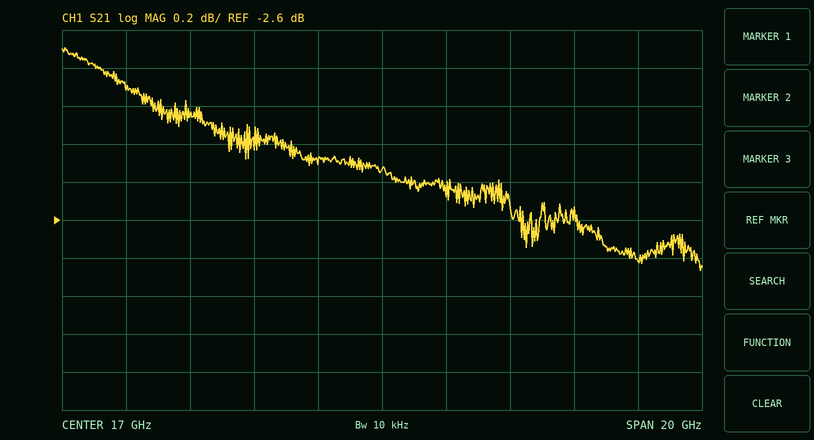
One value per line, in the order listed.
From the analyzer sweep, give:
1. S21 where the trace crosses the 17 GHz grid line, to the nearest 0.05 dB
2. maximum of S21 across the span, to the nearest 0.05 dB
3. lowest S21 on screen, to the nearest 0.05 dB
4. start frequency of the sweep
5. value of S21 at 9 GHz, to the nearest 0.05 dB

-2.35 dB
-1.70 dB
-2.85 dB
7 GHz
-1.90 dB
